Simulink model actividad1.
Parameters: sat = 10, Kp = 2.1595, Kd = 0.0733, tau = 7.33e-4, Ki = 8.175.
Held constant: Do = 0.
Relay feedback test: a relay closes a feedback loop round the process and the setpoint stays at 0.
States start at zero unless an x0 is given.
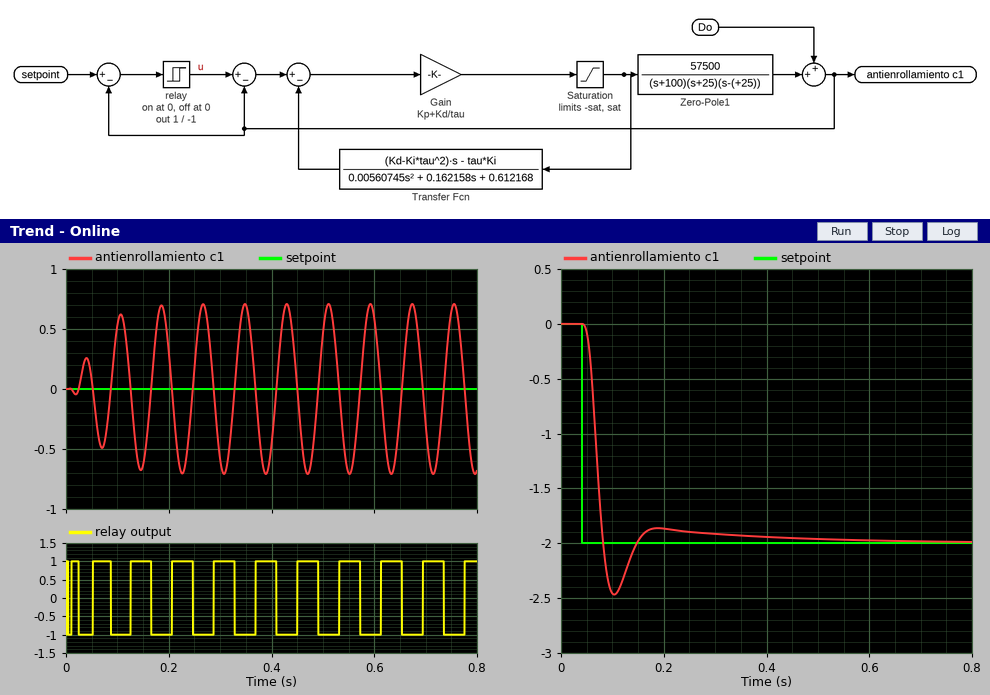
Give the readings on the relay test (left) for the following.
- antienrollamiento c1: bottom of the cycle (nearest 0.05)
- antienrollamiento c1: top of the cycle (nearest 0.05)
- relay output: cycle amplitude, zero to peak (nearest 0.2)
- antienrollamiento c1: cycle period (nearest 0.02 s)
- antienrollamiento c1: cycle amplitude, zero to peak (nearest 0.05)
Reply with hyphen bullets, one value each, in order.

- -0.70
- 0.70
- 1.0
- 0.08 s
- 0.70
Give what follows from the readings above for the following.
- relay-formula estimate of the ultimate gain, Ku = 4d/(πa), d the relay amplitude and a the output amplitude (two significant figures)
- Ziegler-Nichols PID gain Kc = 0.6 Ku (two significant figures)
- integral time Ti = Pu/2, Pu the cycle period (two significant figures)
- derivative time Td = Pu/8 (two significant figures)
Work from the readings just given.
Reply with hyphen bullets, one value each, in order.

- 1.8
- 1.1
- 0.040 s
- 0.010 s
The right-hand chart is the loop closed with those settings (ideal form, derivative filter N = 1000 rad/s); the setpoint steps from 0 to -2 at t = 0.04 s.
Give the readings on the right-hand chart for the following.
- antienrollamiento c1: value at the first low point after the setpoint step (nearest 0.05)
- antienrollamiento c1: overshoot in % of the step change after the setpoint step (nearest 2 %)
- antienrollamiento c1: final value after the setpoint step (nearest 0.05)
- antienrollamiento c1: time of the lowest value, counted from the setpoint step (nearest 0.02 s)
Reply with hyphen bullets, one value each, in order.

- -2.45
- 24 %
- -2.00
- 0.06 s
